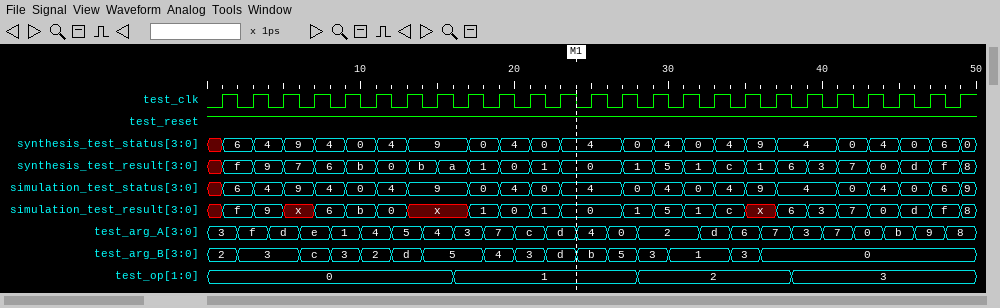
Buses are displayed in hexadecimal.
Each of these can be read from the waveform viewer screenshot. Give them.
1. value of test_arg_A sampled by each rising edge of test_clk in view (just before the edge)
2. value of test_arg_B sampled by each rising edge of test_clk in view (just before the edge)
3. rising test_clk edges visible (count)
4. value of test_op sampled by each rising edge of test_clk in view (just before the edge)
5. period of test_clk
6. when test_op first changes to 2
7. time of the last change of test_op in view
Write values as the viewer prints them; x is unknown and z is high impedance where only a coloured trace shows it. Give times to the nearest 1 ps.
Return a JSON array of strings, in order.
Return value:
["3, f, d, e, 1, 4, 5, 4, 3, 7, c, d, 4, 0, 2, 2, d, 6, 7, 3, 7, 0, b, 9, 8", "2, 3, 3, c, 3, 2, d, 5, 5, 4, 3, d, b, 5, 3, 1, 1, 3, 0, 0, 0, 0, 0, 0, 0", "25", "0, 0, 0, 0, 0, 0, 0, 0, 1, 1, 1, 1, 1, 1, 2, 2, 2, 2, 2, 3, 3, 3, 3, 3, 3", "2 ps", "28 ps", "38 ps"]
